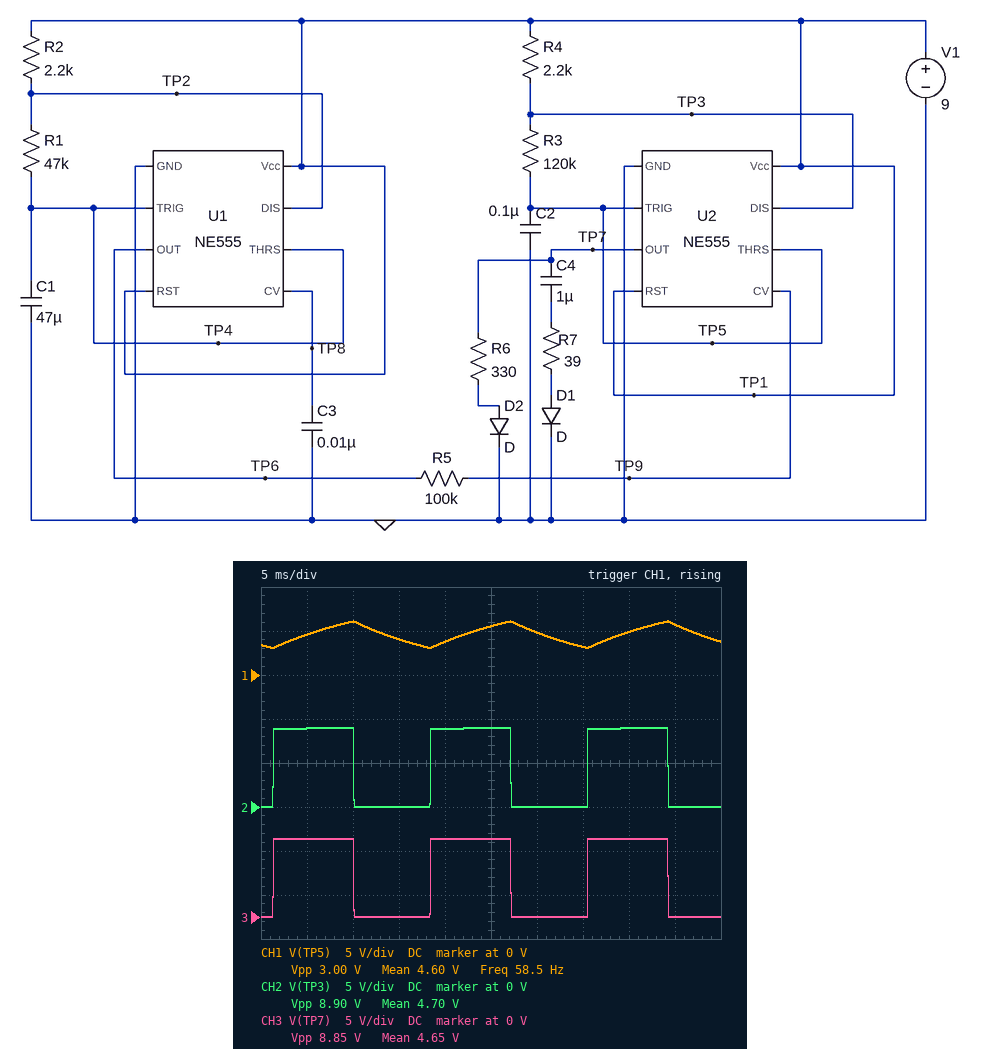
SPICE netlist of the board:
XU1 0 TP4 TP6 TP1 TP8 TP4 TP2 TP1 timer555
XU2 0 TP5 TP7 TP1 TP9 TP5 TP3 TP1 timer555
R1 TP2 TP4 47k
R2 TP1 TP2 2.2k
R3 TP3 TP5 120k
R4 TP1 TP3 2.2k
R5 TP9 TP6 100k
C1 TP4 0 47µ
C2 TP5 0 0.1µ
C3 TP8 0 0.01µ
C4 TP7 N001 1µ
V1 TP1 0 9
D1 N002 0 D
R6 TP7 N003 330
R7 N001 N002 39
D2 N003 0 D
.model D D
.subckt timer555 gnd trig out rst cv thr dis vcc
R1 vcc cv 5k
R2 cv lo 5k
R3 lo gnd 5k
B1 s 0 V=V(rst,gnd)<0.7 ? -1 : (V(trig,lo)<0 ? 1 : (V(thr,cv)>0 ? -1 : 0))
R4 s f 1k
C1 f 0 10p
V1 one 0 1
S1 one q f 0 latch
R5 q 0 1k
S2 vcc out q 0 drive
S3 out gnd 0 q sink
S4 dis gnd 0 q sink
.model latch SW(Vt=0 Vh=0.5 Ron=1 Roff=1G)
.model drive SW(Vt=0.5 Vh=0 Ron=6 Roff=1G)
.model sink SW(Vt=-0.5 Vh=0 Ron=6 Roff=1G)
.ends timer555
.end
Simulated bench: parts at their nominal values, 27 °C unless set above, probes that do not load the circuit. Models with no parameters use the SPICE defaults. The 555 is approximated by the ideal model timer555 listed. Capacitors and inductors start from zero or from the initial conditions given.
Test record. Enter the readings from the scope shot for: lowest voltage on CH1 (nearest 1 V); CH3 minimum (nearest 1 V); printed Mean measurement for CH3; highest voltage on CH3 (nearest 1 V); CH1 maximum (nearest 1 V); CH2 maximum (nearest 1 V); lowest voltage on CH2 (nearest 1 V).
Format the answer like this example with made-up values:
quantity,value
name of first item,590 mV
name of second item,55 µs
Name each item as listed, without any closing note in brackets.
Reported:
quantity,value
lowest voltage on CH1,3 V
CH3 minimum,0 V
printed Mean measurement for CH3,4.65 V
highest voltage on CH3,9 V
CH1 maximum,6 V
CH2 maximum,9 V
lowest voltage on CH2,0 V
